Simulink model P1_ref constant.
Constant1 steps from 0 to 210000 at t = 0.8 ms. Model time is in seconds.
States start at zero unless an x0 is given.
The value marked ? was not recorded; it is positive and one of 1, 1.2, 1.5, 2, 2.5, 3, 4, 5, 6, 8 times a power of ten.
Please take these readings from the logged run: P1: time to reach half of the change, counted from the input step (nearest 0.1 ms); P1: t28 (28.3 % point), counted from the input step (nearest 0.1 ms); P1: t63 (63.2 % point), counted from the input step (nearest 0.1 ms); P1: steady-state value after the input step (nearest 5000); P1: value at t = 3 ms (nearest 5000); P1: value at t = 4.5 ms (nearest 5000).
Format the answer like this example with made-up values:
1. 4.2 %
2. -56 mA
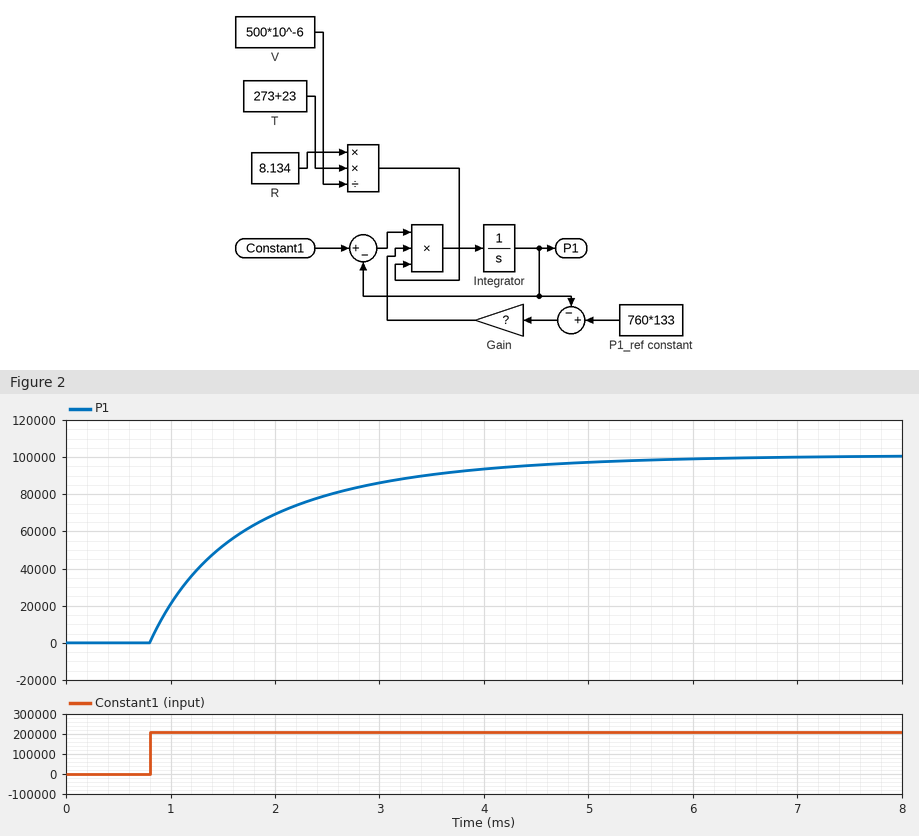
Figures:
1. 0.7 ms
2. 0.3 ms
3. 1.0 ms
4. 100000
5. 85000
6. 95000
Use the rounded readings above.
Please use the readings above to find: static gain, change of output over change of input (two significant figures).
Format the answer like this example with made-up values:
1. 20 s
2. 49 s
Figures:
1. 0.48
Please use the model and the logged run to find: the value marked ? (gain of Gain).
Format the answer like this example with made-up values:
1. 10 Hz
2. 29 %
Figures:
1. 1.2e-09
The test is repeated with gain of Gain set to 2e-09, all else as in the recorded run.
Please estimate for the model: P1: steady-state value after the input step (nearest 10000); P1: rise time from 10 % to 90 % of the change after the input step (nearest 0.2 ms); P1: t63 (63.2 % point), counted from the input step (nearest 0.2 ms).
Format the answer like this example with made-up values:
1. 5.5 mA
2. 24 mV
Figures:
1. 100000
2. 1.6 ms
3. 0.6 ms
